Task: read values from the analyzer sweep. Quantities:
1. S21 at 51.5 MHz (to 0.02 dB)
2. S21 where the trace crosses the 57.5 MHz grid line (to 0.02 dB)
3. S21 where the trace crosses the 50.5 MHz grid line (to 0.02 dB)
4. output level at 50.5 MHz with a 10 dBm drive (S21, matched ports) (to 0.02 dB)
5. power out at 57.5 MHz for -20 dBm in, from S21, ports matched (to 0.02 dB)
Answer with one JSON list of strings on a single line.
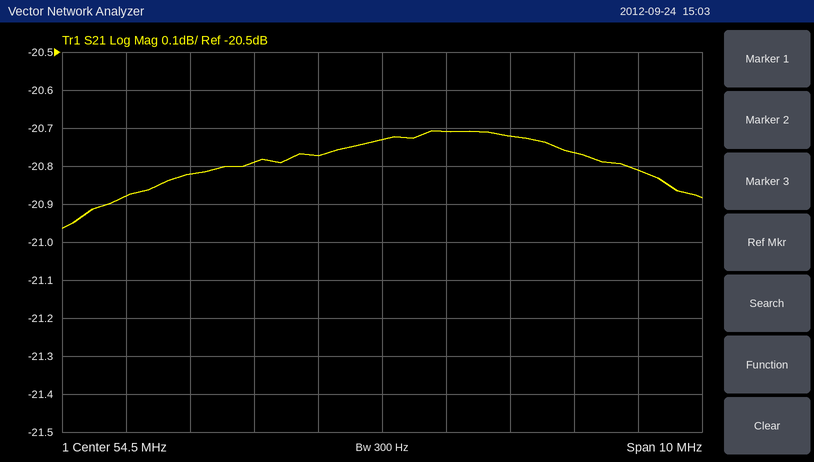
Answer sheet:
["-20.82 dB", "-20.76 dB", "-20.88 dB", "-10.88 dBm", "-40.76 dBm"]
